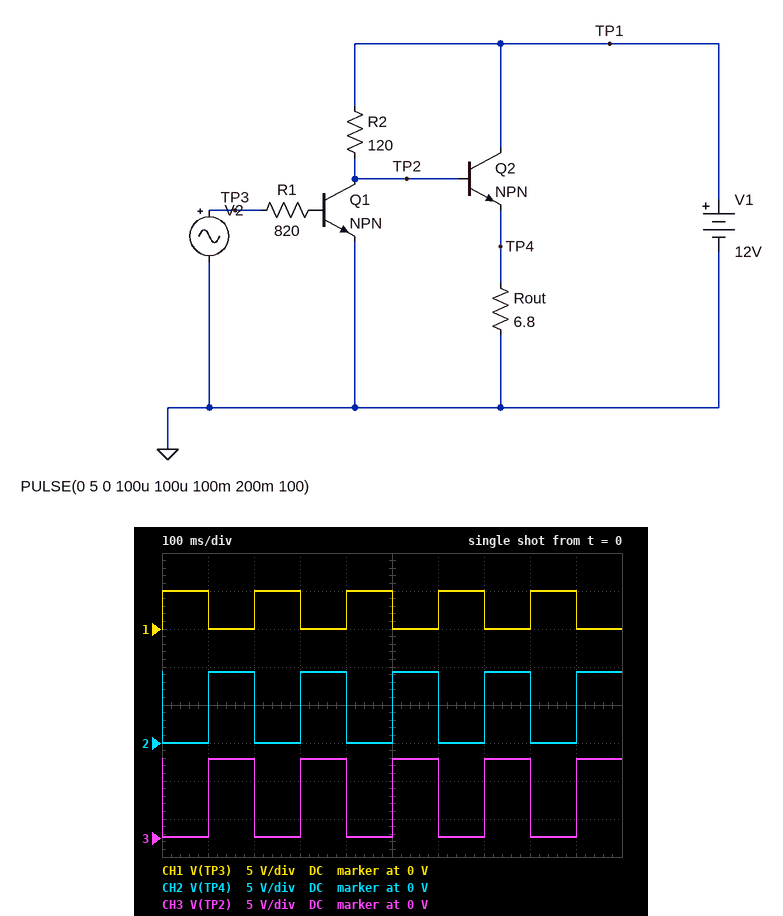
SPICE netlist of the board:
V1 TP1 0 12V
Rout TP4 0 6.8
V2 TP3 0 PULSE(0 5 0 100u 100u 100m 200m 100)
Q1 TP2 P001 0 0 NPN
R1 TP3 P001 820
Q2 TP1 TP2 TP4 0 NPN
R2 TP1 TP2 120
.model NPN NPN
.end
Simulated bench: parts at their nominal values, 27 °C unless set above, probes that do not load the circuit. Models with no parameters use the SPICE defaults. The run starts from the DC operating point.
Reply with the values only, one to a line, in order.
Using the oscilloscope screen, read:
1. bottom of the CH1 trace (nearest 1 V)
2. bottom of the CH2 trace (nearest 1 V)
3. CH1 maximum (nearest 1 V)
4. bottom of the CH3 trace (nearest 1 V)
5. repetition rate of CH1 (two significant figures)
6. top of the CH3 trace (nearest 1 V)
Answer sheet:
0 V
0 V
5 V
0 V
5.0 Hz
10 V
